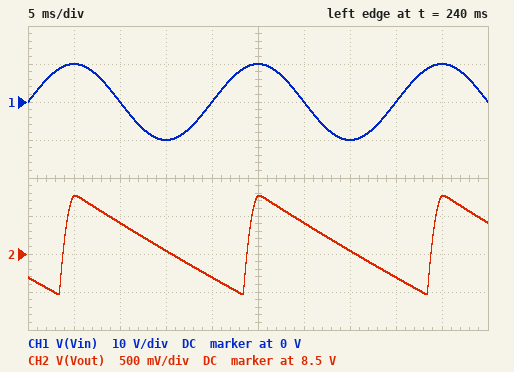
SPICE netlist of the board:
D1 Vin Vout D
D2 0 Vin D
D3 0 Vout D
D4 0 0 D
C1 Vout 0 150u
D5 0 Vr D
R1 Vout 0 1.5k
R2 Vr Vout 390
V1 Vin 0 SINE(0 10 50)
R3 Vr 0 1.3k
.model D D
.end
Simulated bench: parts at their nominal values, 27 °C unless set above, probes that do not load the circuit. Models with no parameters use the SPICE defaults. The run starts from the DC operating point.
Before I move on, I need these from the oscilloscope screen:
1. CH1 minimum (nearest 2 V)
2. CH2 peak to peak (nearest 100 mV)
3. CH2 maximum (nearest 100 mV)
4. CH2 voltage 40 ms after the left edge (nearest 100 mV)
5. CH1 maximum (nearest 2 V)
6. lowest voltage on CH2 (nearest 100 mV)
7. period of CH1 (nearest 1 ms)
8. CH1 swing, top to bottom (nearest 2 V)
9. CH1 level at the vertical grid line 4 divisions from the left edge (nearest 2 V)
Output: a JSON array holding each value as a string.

["-10 V", "1.3 V", "9.3 V", "8.2 V", "10 V", "8.0 V", "20 ms", "20 V", "0 V"]
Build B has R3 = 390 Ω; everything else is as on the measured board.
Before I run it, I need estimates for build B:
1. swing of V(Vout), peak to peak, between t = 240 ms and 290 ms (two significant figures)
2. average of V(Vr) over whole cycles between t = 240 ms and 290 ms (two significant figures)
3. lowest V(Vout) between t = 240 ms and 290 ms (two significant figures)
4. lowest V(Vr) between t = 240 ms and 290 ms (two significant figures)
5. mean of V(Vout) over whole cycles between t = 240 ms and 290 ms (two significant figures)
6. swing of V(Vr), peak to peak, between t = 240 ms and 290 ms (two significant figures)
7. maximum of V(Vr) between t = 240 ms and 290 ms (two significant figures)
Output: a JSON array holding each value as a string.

["1.9 V", "4.2 V", "7.4 V", "3.7 V", "8.3 V", "950 mV", "4.6 V"]
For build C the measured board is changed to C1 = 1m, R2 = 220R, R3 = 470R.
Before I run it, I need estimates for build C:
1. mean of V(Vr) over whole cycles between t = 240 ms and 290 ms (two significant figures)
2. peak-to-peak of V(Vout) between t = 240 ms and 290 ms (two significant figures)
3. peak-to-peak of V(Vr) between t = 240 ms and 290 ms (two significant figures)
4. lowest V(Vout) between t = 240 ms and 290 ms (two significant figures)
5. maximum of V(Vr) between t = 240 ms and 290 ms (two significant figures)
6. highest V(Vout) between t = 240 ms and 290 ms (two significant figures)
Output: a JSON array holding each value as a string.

["6.2 V", "360 mV", "240 mV", "8.9 V", "6.3 V", "9.2 V"]
